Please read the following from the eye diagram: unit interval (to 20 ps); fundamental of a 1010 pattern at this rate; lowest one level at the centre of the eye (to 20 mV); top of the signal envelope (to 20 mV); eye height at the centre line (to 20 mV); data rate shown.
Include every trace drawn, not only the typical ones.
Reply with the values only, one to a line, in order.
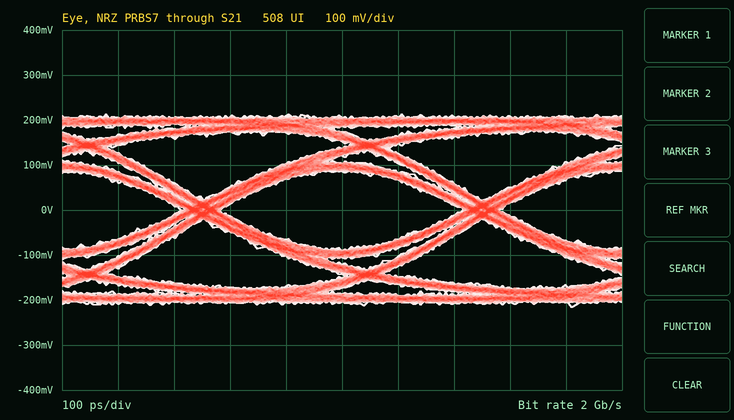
500 ps
1 GHz
80 mV
220 mV
180 mV
2 Gb/s
